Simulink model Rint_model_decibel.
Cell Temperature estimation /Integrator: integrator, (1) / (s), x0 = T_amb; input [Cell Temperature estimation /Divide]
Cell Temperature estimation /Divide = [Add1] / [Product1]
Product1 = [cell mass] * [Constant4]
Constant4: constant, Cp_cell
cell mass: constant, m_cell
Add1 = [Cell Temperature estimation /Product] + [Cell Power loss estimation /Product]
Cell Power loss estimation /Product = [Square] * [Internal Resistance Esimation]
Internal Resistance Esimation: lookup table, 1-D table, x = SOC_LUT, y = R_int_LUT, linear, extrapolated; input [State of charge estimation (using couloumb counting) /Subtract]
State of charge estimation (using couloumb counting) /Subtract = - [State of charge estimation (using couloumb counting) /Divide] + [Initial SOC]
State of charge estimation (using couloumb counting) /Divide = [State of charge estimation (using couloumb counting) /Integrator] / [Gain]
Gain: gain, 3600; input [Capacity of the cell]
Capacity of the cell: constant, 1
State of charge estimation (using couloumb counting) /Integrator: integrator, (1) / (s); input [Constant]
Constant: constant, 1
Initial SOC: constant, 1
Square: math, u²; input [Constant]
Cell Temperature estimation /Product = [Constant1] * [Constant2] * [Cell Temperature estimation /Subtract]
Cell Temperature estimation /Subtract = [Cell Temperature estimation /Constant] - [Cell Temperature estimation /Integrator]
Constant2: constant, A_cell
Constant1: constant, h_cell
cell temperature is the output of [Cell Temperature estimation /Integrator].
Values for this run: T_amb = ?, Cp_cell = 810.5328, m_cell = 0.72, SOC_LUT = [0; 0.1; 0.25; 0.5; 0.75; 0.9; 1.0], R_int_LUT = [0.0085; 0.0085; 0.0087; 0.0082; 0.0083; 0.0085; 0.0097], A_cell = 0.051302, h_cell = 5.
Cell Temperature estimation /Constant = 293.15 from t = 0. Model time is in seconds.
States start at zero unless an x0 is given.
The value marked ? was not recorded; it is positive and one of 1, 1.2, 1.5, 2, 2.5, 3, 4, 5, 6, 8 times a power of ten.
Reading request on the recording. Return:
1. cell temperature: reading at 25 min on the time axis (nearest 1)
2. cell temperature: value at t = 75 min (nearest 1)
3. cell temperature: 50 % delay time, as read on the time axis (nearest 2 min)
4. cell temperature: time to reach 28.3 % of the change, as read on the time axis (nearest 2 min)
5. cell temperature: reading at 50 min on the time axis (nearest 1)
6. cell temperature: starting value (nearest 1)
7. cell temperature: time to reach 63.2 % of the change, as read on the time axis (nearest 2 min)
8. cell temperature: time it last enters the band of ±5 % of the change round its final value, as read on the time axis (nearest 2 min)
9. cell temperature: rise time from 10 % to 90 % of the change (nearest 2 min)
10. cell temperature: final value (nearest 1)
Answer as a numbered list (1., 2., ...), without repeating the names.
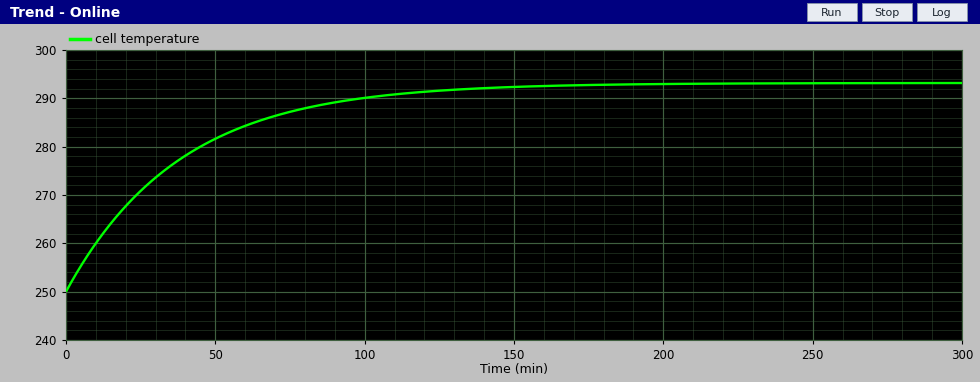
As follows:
1. 271
2. 287
3. 26 min
4. 12 min
5. 282
6. 250
7. 38 min
8. 114 min
9. 84 min
10. 293
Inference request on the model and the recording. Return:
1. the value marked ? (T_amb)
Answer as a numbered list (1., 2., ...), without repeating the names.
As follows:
1. 250
